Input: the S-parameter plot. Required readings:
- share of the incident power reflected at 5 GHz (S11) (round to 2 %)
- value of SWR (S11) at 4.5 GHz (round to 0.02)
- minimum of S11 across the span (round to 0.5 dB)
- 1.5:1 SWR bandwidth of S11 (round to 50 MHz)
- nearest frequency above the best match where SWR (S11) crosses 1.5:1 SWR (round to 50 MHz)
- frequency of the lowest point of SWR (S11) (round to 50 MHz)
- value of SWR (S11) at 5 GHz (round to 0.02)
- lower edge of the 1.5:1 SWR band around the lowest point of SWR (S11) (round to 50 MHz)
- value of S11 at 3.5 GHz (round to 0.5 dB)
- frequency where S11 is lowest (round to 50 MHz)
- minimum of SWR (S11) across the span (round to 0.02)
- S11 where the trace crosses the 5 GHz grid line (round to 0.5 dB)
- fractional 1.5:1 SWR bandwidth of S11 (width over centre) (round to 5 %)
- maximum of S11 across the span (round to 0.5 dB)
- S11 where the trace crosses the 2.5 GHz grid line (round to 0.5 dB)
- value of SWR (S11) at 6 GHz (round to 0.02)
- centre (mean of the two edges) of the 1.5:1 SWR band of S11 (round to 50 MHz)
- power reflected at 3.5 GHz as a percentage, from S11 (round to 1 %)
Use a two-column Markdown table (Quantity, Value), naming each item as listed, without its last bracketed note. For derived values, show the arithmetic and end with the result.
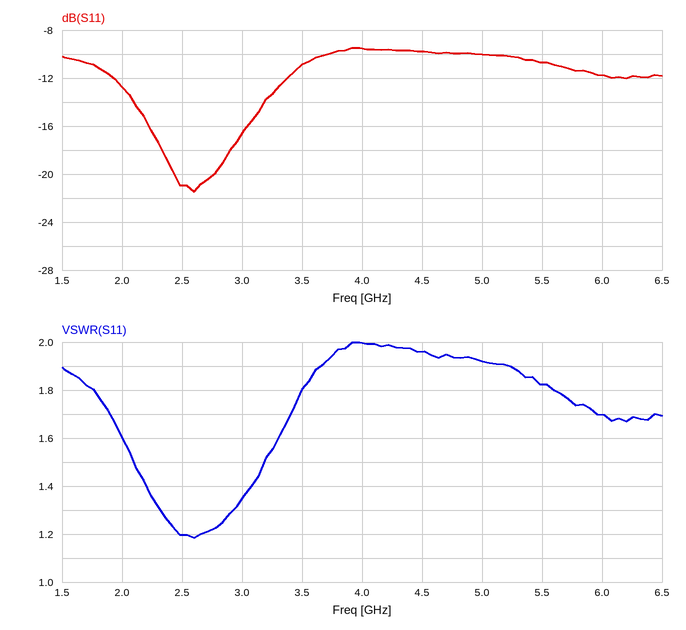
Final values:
| Quantity | Value |
|---|---|
| share of the incident power reflected at 5 GHz (S11) | 10^(-10/10) ≈ 10 % |
| value of SWR (S11) at 4.5 GHz | 1.96 |
| minimum of S11 across the span | -21.5 dB |
| 1.5:1 SWR bandwidth of S11 | 3.20 GHz − 2.10 GHz = 1.10 GHz |
| nearest frequency above the best match where SWR (S11) crosses 1.5:1 SWR | 3.20 GHz |
| frequency of the lowest point of SWR (S11) | 2.60 GHz |
| value of SWR (S11) at 5 GHz | 1.92 |
| lower edge of the 1.5:1 SWR band around the lowest point of SWR (S11) | 2.10 GHz |
| value of S11 at 3.5 GHz | -11.0 dB |
| frequency where S11 is lowest | 2.60 GHz |
| minimum of SWR (S11) across the span | 1.18 |
| S11 where the trace crosses the 5 GHz grid line | -10.0 dB |
| fractional 1.5:1 SWR bandwidth of S11 (width over centre) | 1.1 GHz / 2.65 GHz ≈ 41.5 %, so 40 % to the nearest 5 % |
| maximum of S11 across the span | -9.5 dB |
| S11 where the trace crosses the 2.5 GHz grid line | -21.0 dB |
| value of SWR (S11) at 6 GHz | 1.70 |
| centre (mean of the two edges) of the 1.5:1 SWR band of S11 | 2.65 GHz |
| power reflected at 3.5 GHz as a percentage, from S11 | 10^(-11/10) ≈ 8 % |
